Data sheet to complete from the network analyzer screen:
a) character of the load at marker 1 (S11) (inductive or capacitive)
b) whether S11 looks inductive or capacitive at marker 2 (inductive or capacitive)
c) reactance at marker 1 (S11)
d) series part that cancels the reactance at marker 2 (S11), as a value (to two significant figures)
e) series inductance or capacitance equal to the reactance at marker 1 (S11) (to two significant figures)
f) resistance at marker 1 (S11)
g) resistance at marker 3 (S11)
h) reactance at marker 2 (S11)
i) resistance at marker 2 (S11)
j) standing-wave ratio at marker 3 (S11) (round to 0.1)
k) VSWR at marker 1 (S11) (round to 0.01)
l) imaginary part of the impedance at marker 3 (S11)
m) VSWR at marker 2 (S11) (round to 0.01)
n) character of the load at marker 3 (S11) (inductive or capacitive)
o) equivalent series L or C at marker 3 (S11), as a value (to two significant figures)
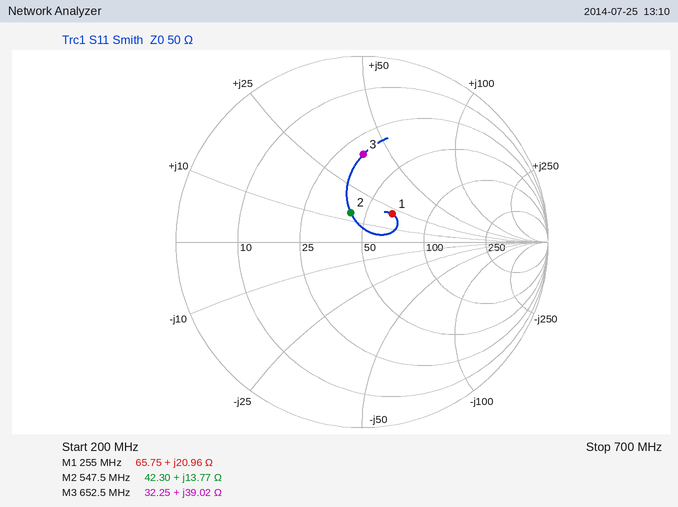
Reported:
inductive
inductive
+20.96 Ω
21 pF
13 nH
65.75 Ω
32.25 Ω
+13.77 Ω
42.30 Ω
2.8
1.57
+39.02 Ω
1.41
inductive
9.5 nH
